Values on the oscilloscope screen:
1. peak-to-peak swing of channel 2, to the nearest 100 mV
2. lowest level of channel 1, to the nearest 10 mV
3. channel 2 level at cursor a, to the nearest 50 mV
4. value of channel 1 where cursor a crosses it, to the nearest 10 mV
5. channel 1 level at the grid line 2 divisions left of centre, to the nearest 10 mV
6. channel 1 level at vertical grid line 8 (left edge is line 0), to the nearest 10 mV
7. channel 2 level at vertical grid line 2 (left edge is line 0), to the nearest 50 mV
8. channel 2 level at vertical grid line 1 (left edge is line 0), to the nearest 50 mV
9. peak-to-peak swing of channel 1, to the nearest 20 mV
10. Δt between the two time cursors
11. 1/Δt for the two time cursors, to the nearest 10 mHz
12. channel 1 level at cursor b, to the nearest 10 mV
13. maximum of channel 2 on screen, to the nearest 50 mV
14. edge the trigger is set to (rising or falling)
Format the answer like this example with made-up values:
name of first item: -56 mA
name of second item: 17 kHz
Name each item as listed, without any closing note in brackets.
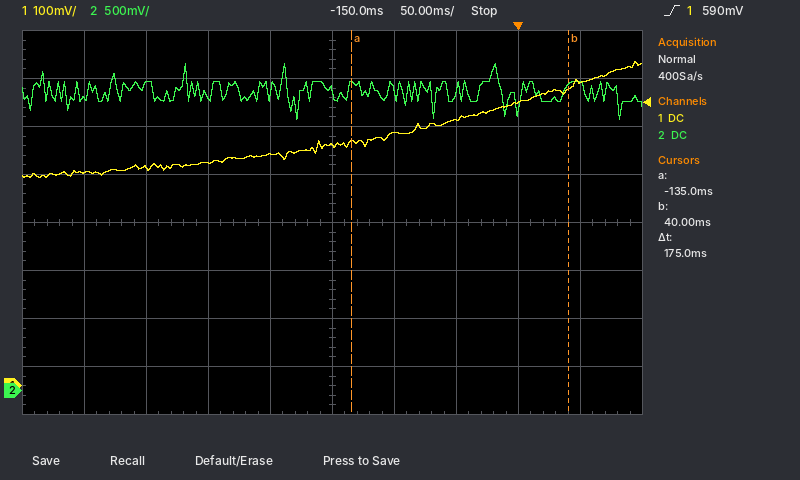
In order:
peak-to-peak swing of channel 2, to the nearest 100 mV: 600 mV
lowest level of channel 1, to the nearest 10 mV: 430 mV
channel 2 level at cursor a, to the nearest 50 mV: 3.15 V
value of channel 1 where cursor a crosses it, to the nearest 10 mV: 510 mV
channel 1 level at the grid line 2 divisions left of centre, to the nearest 10 mV: 460 mV
channel 1 level at vertical grid line 8 (left edge is line 0), to the nearest 10 mV: 590 mV
channel 2 level at vertical grid line 2 (left edge is line 0), to the nearest 50 mV: 3.20 V
channel 2 level at vertical grid line 1 (left edge is line 0), to the nearest 50 mV: 3.05 V
peak-to-peak swing of channel 1, to the nearest 20 mV: 240 mV
Δt between the two time cursors: 175 ms
1/Δt for the two time cursors, to the nearest 10 mHz: 5.71 Hz
channel 1 level at cursor b, to the nearest 10 mV: 620 mV
maximum of channel 2 on screen, to the nearest 50 mV: 3.40 V
edge the trigger is set to: rising
